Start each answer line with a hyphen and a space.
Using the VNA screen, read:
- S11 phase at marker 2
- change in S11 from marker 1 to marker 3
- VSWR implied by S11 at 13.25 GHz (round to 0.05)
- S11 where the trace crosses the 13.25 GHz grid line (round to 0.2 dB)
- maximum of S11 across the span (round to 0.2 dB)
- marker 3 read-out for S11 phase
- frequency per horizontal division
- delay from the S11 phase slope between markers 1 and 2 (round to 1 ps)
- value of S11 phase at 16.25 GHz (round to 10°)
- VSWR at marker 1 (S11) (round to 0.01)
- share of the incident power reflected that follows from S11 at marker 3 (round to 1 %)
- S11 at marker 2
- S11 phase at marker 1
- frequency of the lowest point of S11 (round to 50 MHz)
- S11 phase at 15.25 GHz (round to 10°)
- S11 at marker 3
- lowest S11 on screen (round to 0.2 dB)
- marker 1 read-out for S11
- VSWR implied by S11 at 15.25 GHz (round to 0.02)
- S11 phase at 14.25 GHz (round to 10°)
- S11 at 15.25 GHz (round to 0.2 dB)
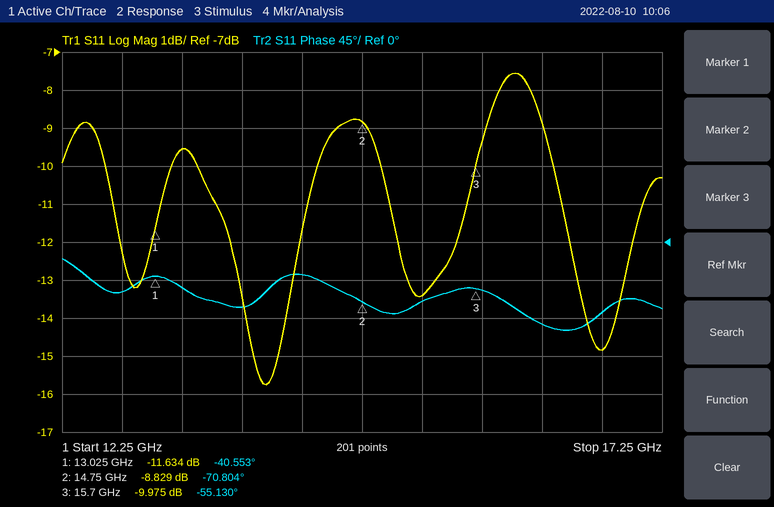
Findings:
- -70.804°
- 1.659 dB
- 2.00
- -9.6 dB
- -7.6 dB
- -55.130°
- 500 MHz
- 49 ps
- -100°
- 1.71
- 10 %
- -8.829 dB
- -40.553°
- 13.95 GHz
- -70°
- -9.975 dB
- -15.8 dB
- -11.634 dB
- 1.54
- -40°
- -13.4 dB
